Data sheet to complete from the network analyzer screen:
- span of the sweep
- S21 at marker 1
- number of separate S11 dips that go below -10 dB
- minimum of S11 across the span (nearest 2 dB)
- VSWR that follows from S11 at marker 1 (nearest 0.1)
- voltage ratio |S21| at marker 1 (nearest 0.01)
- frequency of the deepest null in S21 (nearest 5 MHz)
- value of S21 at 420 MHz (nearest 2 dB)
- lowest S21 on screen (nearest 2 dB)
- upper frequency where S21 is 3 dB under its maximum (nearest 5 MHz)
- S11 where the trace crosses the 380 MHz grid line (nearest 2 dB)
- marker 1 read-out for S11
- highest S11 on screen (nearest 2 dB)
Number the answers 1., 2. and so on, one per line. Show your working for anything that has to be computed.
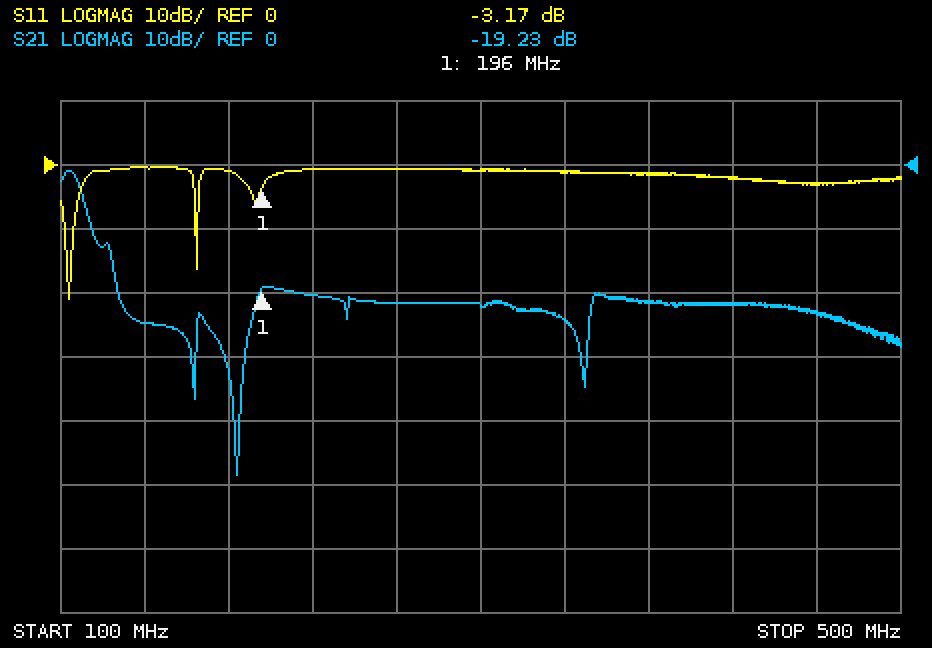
1. 400 MHz
2. -19.23 dB
3. 2
4. -20 dB
5. (1 + 0.6942)/(1 − 0.6942) ≈ 5.5
6. 10^(-19.23/20) ≈ 0.11
7. 185 MHz
8. -22 dB
9. -48 dB
10. 110 MHz
11. -2 dB
12. -3.17 dB
13. 0 dB
